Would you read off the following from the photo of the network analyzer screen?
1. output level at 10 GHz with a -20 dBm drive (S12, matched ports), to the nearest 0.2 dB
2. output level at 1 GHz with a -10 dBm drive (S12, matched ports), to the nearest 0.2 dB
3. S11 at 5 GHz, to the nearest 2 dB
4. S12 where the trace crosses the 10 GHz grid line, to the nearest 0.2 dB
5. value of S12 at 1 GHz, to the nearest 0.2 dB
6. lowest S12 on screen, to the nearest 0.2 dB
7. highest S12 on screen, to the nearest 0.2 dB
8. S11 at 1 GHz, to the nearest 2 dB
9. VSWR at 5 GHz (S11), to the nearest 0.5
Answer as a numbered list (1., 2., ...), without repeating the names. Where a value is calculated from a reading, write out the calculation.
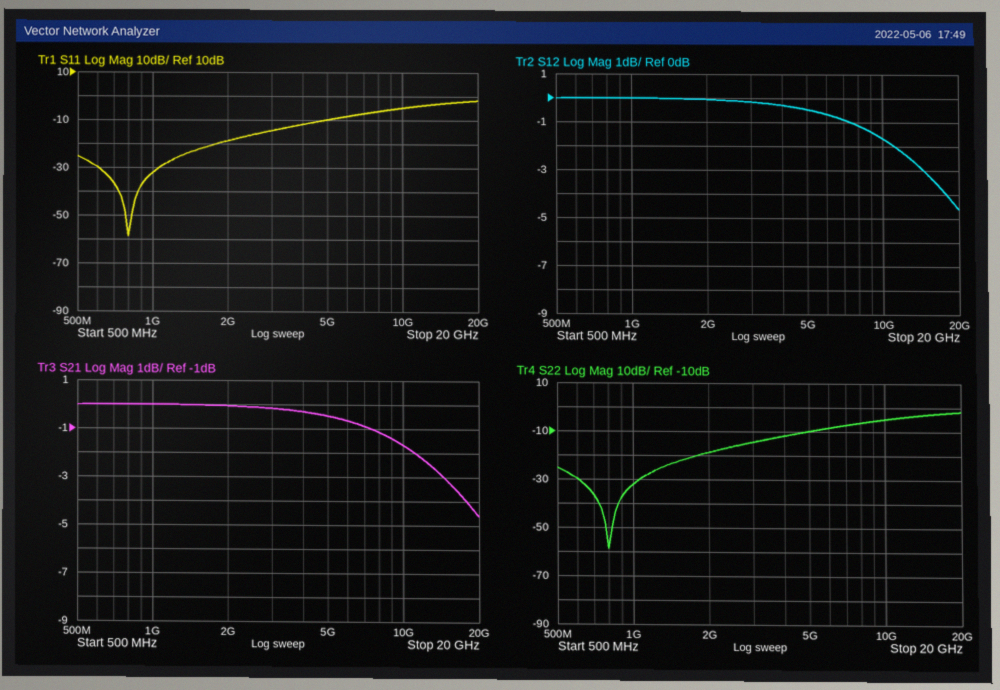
1. -20 dBm + (-1.6 dB) = -21.6 dBm
2. -10 dBm + (0.0 dB) = -10.0 dBm
3. -10 dB
4. -1.6 dB
5. 0.0 dB
6. -4.6 dB
7. 0.0 dB
8. -32 dB
9. |Γ| = 10^(-10/20) = 0.3162; VSWR = (1 + 0.3162)/(1 − 0.3162) ≈ 1.92, so 2.0 to the nearest 0.5
